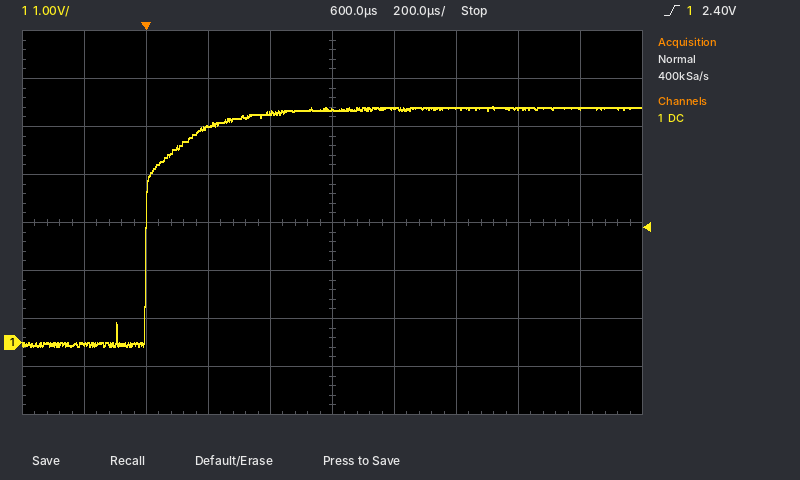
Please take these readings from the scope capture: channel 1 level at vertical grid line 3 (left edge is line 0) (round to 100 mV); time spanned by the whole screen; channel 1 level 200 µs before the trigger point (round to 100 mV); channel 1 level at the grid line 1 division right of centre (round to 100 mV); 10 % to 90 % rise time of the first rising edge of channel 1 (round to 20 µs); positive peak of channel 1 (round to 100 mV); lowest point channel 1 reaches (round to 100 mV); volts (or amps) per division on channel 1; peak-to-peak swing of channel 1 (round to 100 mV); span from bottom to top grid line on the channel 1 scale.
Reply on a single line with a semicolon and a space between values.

4.5 V; 2 ms; 0.0 V; 4.9 V; 180 µs; 4.9 V; -100 mV; 1 V; 5.0 V; 8 V
